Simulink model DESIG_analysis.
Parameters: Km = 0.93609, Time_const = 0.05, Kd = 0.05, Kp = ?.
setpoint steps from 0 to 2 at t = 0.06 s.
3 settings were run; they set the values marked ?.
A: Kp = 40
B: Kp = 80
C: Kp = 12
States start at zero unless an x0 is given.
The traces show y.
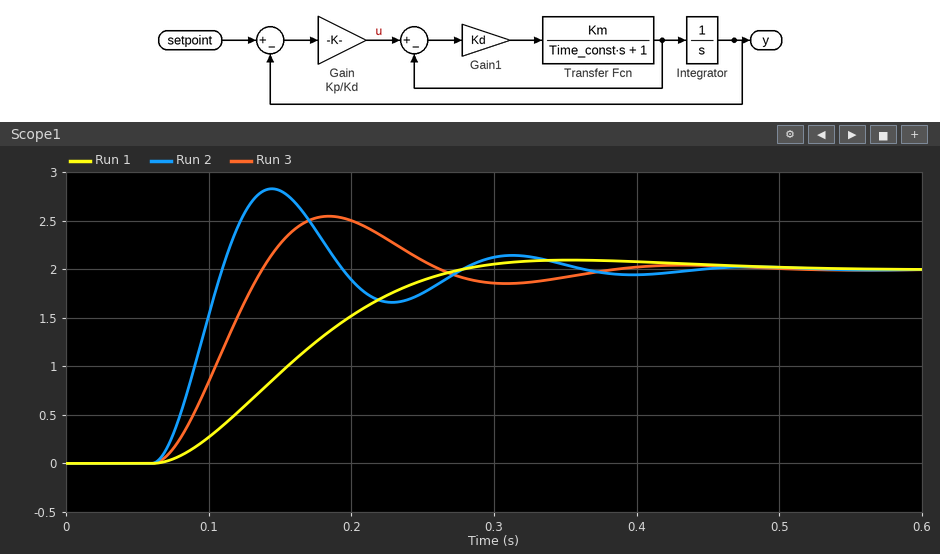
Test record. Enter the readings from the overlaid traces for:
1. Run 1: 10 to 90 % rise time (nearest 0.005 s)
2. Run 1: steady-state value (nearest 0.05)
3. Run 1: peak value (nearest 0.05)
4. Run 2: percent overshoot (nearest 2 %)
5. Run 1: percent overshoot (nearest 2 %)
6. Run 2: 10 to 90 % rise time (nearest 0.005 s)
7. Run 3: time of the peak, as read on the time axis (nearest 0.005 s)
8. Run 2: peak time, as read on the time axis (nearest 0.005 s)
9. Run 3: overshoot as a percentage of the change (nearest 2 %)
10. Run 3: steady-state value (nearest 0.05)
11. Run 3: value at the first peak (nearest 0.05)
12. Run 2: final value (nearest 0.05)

0.140 s
2.00
2.10
42 %
4 %
0.035 s
0.185 s
0.145 s
28 %
2.00
2.55
2.00
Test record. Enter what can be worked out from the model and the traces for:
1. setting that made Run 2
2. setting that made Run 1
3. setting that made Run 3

B
C
A
